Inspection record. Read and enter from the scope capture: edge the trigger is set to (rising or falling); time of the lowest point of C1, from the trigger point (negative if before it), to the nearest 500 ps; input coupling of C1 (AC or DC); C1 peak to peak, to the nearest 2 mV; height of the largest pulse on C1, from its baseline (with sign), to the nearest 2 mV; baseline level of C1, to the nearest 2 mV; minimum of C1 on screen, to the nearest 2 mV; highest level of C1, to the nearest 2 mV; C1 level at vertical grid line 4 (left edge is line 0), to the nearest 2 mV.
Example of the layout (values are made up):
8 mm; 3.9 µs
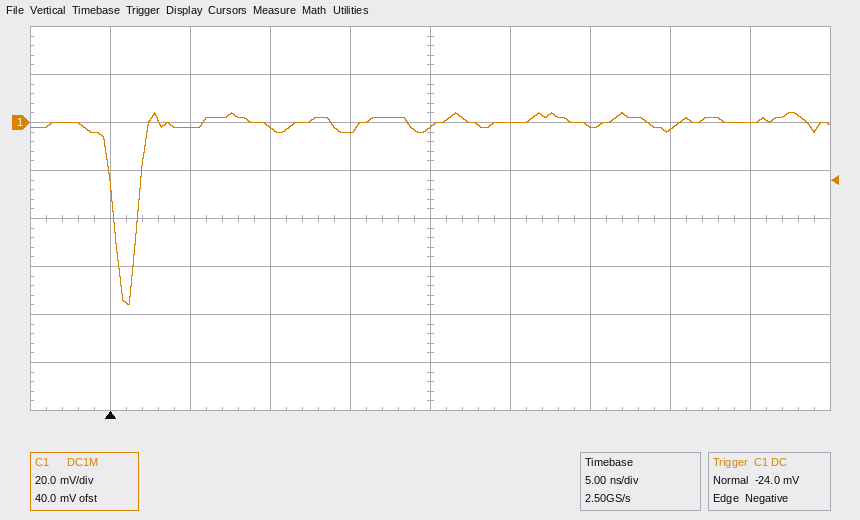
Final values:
falling; +1.0 ns; DC; 80 mV; -76 mV; 0 mV; -76 mV; 4 mV; -4 mV
